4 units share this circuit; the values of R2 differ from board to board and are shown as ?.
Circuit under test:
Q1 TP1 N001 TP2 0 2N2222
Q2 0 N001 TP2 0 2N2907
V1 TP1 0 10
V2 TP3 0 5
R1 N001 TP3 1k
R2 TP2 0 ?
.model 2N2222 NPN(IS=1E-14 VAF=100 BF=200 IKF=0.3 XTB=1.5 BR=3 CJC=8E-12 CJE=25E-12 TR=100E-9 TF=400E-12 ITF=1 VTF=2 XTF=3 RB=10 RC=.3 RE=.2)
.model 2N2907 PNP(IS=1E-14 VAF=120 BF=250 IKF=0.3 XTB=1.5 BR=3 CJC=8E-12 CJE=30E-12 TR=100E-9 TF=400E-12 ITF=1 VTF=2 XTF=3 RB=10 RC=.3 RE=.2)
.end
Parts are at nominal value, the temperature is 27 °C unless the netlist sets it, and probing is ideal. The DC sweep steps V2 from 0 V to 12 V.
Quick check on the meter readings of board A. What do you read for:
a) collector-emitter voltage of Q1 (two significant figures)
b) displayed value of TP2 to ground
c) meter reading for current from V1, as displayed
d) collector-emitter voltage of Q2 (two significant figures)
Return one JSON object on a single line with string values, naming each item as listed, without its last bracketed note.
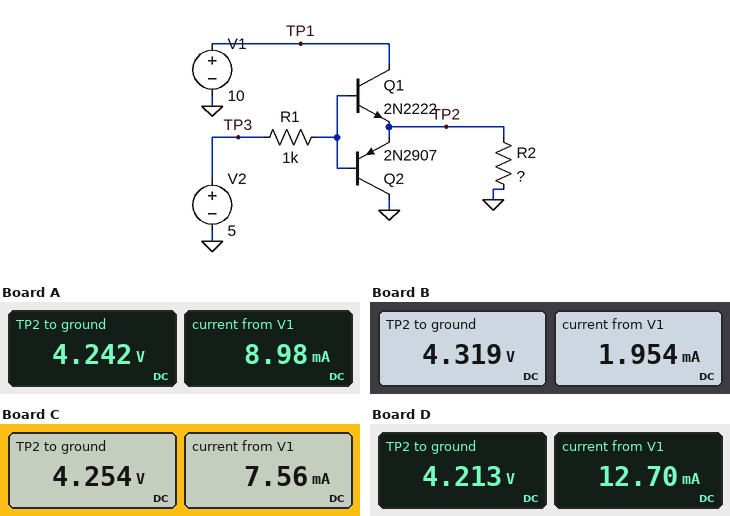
{"collector-emitter voltage of Q1": "5.8 V", "displayed value of TP2 to ground": "4.242 V", "meter reading for current from V1, as displayed": "8.98 mA", "collector-emitter voltage of Q2": "-4.2 V"}
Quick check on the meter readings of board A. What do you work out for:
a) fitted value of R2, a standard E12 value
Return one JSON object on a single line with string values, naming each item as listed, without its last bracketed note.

{"fitted value of R2, a standard E12 value": "470 Ω"}
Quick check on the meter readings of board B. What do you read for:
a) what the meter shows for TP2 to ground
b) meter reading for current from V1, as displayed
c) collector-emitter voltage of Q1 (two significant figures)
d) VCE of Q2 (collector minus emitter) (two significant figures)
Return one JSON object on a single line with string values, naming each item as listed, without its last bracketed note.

{"what the meter shows for TP2 to ground": "4.319 V", "meter reading for current from V1, as displayed": "1.954 mA", "collector-emitter voltage of Q1": "5.7 V", "VCE of Q2 (collector minus emitter)": "-4.3 V"}
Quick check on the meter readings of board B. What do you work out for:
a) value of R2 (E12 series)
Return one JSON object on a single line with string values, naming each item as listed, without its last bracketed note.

{"value of R2": "2.2 kΩ"}
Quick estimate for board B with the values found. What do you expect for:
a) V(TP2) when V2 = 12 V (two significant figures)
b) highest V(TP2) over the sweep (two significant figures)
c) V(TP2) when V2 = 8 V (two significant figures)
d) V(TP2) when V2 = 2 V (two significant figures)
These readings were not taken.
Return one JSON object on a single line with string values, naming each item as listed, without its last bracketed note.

{"V(TP2) when V2 = 12 V": "10 V", "highest V(TP2) over the sweep": "10 V", "V(TP2) when V2 = 8 V": "7.3 V", "V(TP2) when V2 = 2 V": "1.4 V"}
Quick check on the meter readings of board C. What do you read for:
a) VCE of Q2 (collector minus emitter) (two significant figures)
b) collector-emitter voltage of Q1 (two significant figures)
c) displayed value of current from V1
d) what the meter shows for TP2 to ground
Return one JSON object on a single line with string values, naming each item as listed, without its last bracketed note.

{"VCE of Q2 (collector minus emitter)": "-4.3 V", "collector-emitter voltage of Q1": "5.7 V", "displayed value of current from V1": "7.56 mA", "what the meter shows for TP2 to ground": "4.254 V"}
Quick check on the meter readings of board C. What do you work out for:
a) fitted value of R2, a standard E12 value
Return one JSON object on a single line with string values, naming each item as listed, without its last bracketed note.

{"fitted value of R2, a standard E12 value": "560 Ω"}
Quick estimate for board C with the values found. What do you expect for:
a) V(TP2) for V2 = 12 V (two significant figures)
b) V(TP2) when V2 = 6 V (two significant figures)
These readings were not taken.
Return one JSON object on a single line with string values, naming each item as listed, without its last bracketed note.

{"V(TP2) for V2 = 12 V": "9.9 V", "V(TP2) when V2 = 6 V": "5.2 V"}
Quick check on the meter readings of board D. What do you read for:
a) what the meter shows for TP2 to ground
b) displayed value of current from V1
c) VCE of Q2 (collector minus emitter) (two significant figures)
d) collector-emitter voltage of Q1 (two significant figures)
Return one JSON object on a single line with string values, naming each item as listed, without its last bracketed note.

{"what the meter shows for TP2 to ground": "4.213 V", "displayed value of current from V1": "12.70 mA", "VCE of Q2 (collector minus emitter)": "-4.2 V", "collector-emitter voltage of Q1": "5.8 V"}
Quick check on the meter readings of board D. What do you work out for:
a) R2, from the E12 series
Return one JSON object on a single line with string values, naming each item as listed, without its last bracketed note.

{"R2, from the E12 series": "330 Ω"}
